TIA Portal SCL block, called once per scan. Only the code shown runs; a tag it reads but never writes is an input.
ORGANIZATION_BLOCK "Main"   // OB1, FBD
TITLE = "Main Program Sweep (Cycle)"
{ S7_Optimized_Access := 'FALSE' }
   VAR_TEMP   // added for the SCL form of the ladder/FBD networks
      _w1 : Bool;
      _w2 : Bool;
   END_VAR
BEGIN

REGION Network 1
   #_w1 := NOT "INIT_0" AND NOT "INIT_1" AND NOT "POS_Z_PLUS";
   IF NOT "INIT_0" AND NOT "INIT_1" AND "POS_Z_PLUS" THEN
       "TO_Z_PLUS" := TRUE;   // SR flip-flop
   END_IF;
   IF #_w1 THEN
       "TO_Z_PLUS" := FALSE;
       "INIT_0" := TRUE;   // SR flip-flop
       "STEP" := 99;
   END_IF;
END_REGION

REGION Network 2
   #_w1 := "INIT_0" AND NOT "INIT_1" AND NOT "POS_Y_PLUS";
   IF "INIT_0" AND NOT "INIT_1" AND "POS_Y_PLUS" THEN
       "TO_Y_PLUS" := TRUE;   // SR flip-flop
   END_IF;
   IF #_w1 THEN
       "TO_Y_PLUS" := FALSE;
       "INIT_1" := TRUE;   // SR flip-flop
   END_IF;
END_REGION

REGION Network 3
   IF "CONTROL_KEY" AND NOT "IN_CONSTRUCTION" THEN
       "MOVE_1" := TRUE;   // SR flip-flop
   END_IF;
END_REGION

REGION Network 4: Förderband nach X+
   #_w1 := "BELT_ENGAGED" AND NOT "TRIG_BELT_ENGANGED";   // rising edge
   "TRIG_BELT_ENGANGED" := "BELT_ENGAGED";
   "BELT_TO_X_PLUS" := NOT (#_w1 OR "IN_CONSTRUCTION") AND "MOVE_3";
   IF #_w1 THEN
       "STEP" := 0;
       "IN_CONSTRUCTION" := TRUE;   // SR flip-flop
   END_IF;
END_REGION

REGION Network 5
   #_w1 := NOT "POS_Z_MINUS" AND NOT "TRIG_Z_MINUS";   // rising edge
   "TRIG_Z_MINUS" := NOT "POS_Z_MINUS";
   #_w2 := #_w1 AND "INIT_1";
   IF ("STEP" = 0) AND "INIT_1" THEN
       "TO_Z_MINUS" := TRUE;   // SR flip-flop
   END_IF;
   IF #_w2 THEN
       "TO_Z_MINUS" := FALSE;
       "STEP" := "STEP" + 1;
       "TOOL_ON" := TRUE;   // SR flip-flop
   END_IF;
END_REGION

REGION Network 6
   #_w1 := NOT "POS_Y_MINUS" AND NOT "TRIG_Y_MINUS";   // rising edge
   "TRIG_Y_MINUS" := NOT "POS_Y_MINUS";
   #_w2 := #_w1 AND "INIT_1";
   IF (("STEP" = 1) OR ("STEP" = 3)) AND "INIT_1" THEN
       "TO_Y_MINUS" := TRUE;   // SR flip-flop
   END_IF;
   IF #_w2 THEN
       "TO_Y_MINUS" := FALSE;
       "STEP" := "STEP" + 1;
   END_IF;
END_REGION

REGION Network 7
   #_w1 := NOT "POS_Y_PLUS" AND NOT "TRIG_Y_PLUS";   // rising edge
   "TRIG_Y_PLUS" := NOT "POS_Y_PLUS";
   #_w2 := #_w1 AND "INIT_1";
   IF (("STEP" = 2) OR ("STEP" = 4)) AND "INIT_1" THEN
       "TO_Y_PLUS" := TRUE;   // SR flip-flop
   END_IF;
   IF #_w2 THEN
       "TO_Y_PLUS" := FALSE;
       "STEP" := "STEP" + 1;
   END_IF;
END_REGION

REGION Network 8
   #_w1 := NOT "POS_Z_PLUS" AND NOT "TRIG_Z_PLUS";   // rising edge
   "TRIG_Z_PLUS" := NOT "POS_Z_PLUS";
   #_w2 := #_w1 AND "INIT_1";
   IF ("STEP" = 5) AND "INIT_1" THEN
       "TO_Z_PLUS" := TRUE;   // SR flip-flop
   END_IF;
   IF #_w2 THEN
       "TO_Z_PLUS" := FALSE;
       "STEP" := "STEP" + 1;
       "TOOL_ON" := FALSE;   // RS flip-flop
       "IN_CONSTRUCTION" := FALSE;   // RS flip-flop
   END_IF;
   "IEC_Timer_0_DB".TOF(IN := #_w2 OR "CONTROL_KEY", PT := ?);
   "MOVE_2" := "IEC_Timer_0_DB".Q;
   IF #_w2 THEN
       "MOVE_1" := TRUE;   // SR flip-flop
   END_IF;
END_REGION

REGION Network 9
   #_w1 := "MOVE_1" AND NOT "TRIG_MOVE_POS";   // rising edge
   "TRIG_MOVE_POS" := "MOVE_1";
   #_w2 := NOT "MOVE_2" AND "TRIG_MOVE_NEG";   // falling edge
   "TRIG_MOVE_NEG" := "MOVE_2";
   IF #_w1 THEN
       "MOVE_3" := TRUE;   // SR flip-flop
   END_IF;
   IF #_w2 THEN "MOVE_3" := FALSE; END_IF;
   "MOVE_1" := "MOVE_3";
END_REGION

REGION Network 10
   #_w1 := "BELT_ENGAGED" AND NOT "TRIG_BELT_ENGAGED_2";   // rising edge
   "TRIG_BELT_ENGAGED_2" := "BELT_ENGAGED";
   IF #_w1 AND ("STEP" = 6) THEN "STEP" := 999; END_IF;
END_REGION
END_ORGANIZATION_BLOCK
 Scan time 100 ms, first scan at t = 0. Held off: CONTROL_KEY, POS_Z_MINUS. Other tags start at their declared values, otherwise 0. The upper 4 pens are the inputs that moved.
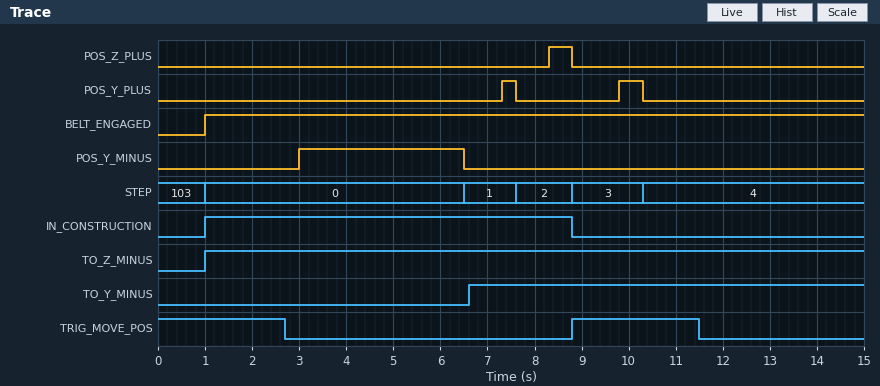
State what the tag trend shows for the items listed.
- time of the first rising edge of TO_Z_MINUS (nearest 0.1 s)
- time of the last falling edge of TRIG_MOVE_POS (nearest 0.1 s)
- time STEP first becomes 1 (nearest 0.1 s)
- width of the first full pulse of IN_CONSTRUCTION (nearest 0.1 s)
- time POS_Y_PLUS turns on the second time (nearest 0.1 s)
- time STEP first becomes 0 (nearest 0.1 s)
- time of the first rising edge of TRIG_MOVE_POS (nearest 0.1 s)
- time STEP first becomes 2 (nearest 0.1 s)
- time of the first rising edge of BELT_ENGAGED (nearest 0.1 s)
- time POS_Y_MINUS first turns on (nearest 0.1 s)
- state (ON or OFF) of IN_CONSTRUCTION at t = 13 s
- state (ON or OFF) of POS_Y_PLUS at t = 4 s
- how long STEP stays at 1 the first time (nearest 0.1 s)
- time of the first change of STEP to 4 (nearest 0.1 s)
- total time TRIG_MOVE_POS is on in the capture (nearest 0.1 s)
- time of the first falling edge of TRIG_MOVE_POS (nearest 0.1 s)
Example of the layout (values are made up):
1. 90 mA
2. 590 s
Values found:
1. 1.0 s
2. 11.5 s
3. 6.5 s
4. 7.8 s
5. 9.8 s
6. 1.0 s
7. 8.8 s
8. 7.6 s
9. 1.0 s
10. 3.0 s
11. OFF
12. OFF
13. 1.1 s
14. 10.3 s
15. 5.4 s
16. 2.7 s
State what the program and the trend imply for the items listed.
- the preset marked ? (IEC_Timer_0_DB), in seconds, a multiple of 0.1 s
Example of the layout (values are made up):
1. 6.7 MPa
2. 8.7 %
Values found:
1. 2.5 s
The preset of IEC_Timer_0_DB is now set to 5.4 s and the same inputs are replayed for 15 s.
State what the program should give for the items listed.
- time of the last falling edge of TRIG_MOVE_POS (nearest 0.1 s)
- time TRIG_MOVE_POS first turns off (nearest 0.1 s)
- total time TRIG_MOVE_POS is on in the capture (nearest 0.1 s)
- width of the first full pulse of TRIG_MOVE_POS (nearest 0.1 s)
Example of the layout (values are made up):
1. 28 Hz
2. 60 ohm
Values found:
1. 14.4 s
2. 5.6 s
3. 11.2 s
4. 5.6 s
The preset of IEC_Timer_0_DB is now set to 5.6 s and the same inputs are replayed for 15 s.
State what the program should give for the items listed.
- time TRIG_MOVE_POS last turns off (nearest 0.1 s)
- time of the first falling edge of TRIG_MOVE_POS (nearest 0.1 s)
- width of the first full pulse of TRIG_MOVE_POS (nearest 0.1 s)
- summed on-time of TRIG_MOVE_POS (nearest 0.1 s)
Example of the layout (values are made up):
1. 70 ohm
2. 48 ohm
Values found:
1. 14.6 s
2. 5.8 s
3. 5.8 s
4. 11.6 s
